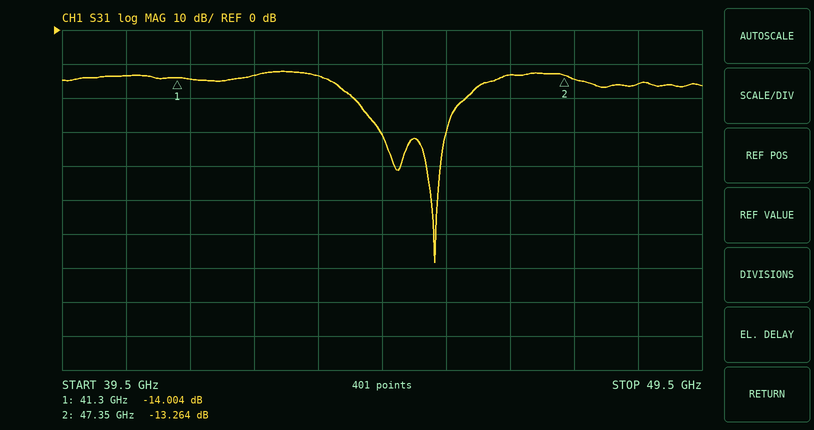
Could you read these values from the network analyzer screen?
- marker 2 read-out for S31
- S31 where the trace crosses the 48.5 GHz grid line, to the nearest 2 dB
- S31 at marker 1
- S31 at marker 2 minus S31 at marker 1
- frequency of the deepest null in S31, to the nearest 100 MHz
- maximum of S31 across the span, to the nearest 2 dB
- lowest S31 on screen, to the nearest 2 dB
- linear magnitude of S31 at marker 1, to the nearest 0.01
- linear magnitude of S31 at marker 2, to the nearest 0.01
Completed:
-13.264 dB
-16 dB
-14.004 dB
0.740 dB
45.3 GHz
-12 dB
-68 dB
0.20
0.22
